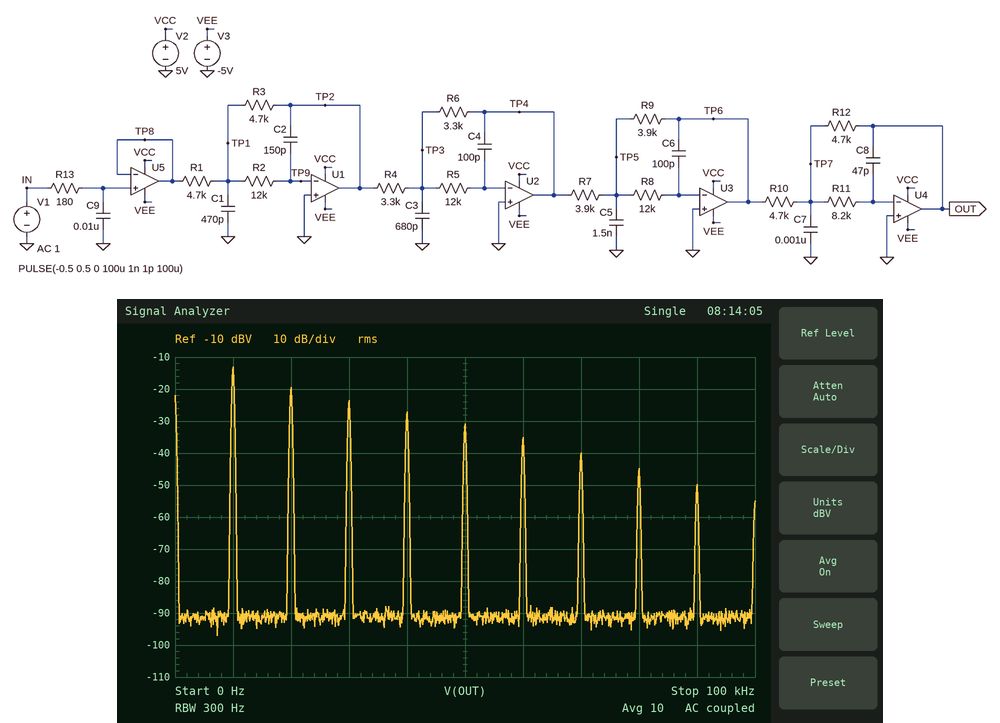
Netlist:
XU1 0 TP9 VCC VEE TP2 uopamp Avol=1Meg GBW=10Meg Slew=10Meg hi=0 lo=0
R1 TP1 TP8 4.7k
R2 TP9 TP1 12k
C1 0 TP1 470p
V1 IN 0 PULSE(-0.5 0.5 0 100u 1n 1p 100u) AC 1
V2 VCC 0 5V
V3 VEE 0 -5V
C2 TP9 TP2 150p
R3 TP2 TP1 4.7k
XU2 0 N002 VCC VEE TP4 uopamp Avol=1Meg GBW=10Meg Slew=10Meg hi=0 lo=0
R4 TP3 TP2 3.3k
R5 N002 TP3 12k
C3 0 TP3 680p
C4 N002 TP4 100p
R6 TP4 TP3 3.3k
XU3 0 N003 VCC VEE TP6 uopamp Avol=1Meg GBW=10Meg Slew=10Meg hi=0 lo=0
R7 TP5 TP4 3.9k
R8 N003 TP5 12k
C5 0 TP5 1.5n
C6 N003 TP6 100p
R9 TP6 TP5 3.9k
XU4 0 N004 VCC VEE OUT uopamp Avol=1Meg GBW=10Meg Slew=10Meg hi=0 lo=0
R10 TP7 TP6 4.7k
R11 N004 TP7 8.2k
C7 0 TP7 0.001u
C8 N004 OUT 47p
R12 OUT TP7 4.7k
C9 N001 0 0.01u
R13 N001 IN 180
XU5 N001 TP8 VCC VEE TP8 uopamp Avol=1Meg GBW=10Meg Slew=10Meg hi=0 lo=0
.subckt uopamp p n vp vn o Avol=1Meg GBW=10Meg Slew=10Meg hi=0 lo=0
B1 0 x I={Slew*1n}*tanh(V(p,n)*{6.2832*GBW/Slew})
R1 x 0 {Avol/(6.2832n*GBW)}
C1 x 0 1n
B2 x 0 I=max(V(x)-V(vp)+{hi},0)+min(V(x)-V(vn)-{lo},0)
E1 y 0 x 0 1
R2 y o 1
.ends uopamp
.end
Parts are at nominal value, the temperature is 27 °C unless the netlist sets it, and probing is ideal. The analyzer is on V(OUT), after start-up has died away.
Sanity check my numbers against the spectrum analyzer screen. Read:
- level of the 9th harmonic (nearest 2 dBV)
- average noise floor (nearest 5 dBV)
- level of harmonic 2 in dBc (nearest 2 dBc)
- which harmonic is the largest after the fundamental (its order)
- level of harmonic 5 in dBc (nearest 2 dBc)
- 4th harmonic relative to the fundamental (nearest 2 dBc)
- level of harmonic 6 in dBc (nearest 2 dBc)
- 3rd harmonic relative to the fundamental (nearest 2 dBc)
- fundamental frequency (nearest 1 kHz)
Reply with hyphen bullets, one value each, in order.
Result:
- -50 dBV
- -90 dBV
- -6 dBc
- 2
- -18 dBc
- -14 dBc
- -22 dBc
- -10 dBc
- 10 kHz
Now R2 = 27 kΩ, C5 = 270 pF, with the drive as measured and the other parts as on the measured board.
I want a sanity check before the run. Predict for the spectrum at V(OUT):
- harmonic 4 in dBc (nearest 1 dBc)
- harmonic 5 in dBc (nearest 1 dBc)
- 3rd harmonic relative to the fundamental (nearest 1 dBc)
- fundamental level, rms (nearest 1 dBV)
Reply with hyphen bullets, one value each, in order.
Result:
- -20 dBc
- -25 dBc
- -15 dBc
- -14 dBV
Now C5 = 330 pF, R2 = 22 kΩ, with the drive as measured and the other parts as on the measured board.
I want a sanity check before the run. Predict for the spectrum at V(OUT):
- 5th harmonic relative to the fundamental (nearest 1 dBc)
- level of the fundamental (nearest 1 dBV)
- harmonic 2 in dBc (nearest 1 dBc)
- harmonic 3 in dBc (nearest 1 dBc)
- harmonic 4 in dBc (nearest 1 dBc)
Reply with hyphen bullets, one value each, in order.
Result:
- -23 dBc
- -14 dBV
- -8 dBc
- -14 dBc
- -19 dBc
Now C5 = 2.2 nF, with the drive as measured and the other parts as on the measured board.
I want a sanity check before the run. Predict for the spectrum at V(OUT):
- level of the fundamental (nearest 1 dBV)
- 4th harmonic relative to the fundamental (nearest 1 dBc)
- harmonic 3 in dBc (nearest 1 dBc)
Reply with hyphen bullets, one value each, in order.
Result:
- -13 dBV
- -13 dBc
- -10 dBc
